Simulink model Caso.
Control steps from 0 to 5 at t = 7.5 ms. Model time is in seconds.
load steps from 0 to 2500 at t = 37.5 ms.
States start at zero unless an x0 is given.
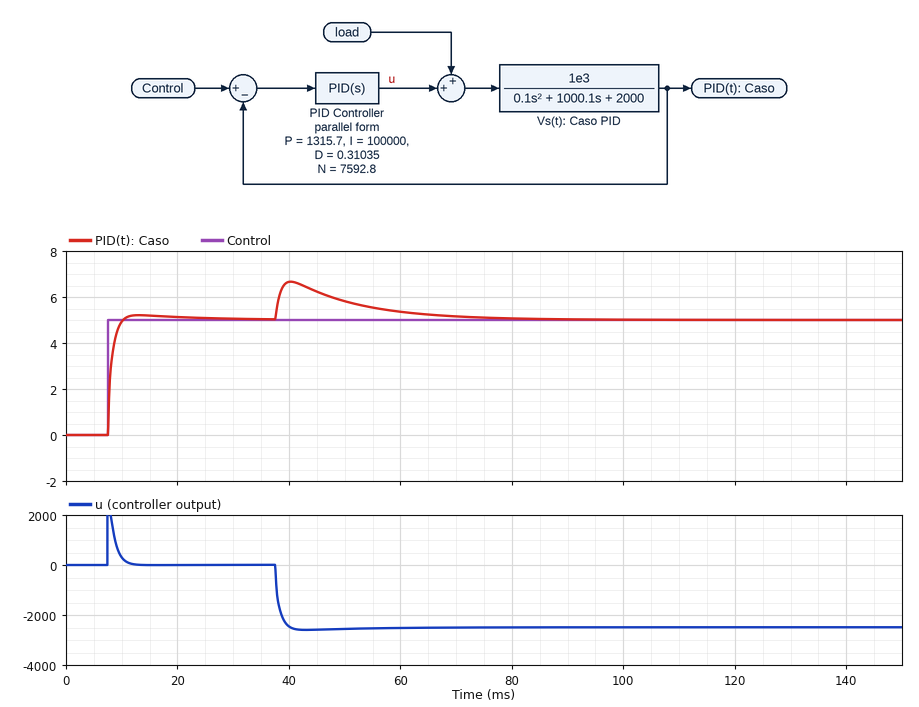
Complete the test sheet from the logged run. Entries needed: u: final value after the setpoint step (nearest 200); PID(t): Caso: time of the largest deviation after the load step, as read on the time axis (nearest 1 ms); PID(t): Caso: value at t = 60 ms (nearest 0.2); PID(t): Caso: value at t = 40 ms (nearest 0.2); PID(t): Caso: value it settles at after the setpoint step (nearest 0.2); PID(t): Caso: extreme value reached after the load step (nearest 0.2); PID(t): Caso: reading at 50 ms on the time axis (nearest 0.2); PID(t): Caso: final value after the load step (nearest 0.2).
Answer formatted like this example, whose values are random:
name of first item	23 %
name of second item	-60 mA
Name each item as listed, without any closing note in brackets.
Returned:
u: final value after the setpoint step	0
PID(t): Caso: time of the largest deviation after the load step, as read on the time axis	40 ms
PID(t): Caso: value at t = 60 ms	5.4
PID(t): Caso: value at t = 40 ms	6.6
PID(t): Caso: value it settles at after the setpoint step	5.0
PID(t): Caso: extreme value reached after the load step	6.6
PID(t): Caso: reading at 50 ms on the time axis	5.8
PID(t): Caso: final value after the load step	5.0
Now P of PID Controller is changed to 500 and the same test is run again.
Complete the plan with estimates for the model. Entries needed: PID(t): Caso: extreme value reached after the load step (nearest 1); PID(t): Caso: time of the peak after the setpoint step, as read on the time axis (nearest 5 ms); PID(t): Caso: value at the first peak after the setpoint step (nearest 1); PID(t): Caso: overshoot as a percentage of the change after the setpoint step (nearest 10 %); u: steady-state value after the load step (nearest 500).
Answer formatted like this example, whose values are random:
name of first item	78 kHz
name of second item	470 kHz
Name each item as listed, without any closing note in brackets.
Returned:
PID(t): Caso: extreme value reached after the load step	8
PID(t): Caso: time of the peak after the setpoint step, as read on the time axis	15 ms
PID(t): Caso: value at the first peak after the setpoint step	6
PID(t): Caso: overshoot as a percentage of the change after the setpoint step	20 %
u: steady-state value after the load step	-2500
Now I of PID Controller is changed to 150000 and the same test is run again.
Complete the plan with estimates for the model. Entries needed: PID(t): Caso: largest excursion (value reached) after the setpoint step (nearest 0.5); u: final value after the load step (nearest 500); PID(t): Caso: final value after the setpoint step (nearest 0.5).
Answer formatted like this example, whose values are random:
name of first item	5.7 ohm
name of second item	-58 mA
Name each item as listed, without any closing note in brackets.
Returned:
PID(t): Caso: largest excursion (value reached) after the setpoint step	5.5
u: final value after the load step	-2500
PID(t): Caso: final value after the setpoint step	5.0
